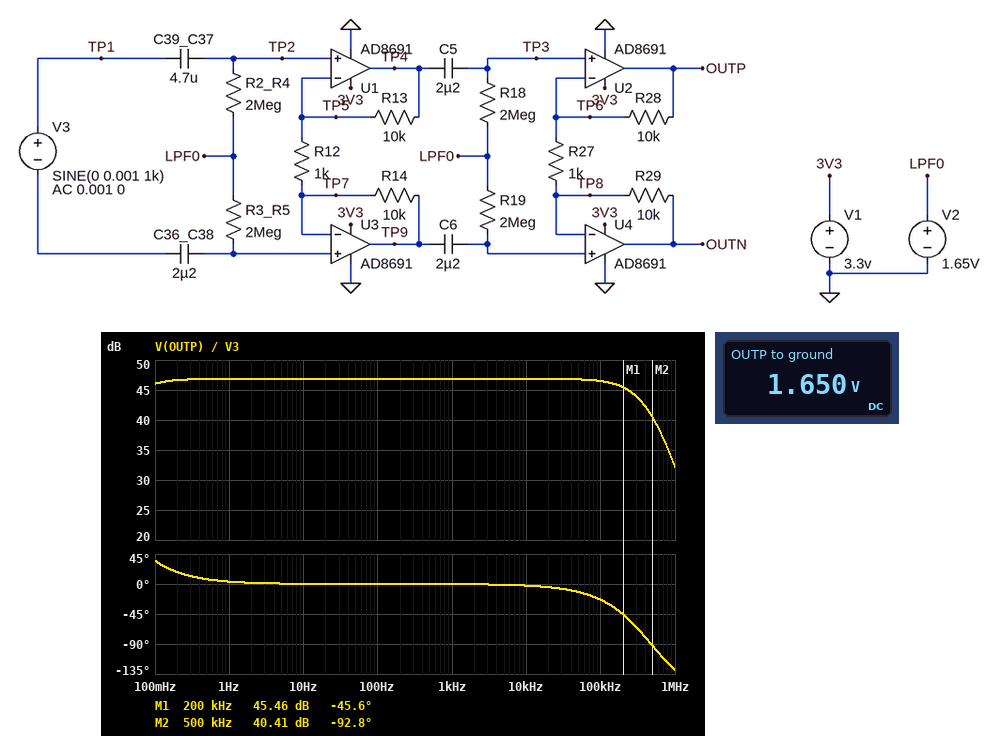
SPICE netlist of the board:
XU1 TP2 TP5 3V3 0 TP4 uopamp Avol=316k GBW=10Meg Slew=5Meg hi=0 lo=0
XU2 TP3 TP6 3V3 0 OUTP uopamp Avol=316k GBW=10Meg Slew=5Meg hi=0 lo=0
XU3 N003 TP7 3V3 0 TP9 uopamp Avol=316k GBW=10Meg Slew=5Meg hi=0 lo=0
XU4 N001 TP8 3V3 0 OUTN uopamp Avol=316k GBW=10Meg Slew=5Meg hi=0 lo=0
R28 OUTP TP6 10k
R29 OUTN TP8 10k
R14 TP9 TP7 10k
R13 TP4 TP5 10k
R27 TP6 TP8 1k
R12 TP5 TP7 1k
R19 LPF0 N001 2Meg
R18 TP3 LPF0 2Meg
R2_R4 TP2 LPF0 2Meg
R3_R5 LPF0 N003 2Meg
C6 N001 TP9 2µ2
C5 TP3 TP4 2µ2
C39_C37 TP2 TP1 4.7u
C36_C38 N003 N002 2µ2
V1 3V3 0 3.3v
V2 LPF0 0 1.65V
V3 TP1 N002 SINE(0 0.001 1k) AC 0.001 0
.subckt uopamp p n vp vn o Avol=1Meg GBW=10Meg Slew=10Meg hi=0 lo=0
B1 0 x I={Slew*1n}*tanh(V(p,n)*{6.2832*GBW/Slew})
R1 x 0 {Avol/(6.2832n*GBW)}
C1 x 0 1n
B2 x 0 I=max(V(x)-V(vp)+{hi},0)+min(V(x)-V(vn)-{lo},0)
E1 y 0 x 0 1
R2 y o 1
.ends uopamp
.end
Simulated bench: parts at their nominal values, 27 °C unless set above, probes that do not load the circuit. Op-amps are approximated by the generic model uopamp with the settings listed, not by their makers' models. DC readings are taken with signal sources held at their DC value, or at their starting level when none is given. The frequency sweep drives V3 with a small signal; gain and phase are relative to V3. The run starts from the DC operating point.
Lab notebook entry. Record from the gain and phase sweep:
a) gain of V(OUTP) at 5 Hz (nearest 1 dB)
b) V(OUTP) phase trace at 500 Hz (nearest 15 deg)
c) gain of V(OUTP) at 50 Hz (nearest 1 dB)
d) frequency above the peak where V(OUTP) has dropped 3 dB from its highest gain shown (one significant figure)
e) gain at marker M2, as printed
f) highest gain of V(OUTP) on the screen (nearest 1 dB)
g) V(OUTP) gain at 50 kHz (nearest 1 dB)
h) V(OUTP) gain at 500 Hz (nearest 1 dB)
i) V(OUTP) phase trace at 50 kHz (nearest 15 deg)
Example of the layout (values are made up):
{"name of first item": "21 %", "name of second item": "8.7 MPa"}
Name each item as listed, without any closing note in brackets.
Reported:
{"gain of V(OUTP) at 5 Hz": "47 dB", "V(OUTP) phase trace at 500 Hz": "0 deg", "gain of V(OUTP) at 50 Hz": "47 dB", "frequency above the peak where V(OUTP) has dropped 3 dB from its highest gain shown": "300 kHz", "gain at marker M2, as printed": "40.41 dB", "highest gain of V(OUTP) on the screen": "47 dB", "V(OUTP) gain at 50 kHz": "47 dB", "V(OUTP) gain at 500 Hz": "47 dB", "V(OUTP) phase trace at 50 kHz": "-15 deg"}
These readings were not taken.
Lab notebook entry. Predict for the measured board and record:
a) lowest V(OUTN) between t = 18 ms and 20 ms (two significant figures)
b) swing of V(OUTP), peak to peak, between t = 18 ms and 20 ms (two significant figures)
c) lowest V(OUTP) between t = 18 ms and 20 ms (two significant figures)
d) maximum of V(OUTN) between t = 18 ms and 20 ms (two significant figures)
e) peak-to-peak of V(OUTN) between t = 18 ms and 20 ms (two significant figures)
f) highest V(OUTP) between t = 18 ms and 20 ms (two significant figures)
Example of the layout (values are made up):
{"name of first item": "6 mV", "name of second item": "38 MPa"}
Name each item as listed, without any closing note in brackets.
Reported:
{"lowest V(OUTN) between t = 18 ms and 20 ms": "1.4 V", "swing of V(OUTP), peak to peak, between t = 18 ms and 20 ms": "440 mV", "lowest V(OUTP) between t = 18 ms and 20 ms": "1.4 V", "maximum of V(OUTN) between t = 18 ms and 20 ms": "1.9 V", "peak-to-peak of V(OUTN) between t = 18 ms and 20 ms": "440 mV", "highest V(OUTP) between t = 18 ms and 20 ms": "1.9 V"}
